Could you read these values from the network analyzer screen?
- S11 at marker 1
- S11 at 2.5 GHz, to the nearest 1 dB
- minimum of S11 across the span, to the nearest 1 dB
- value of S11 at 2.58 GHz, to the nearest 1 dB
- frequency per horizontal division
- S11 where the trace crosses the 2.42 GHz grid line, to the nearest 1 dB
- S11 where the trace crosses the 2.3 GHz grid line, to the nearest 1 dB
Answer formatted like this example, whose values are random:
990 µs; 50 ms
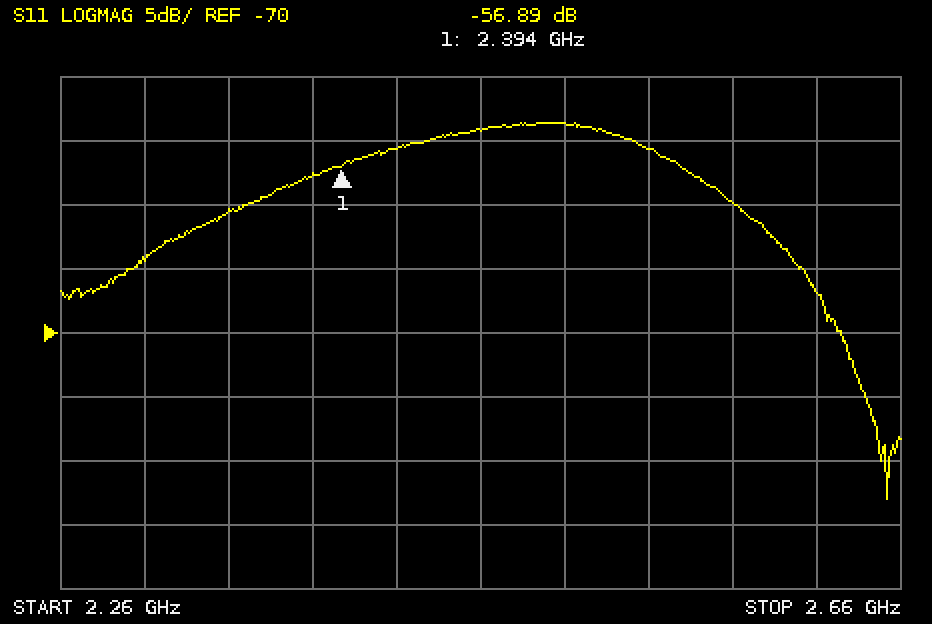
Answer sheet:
-56.89 dB; -54 dB; -83 dB; -60 dB; 40 MHz; -56 dB; -64 dB
